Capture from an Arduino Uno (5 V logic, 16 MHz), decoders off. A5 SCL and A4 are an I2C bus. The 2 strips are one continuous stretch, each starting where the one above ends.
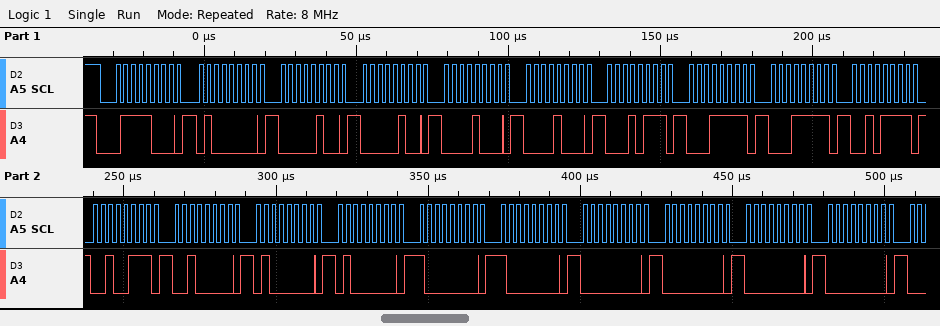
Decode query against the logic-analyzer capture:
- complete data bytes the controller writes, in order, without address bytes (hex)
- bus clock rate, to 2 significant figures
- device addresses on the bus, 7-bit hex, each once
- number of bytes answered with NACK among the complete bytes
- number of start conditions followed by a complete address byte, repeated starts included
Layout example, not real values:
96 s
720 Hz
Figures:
40 04 04 08 08 17 1F 1F 2F 27 20 40 40 80 80 00 00 00 00
400 kHz
0x3C
0
1
